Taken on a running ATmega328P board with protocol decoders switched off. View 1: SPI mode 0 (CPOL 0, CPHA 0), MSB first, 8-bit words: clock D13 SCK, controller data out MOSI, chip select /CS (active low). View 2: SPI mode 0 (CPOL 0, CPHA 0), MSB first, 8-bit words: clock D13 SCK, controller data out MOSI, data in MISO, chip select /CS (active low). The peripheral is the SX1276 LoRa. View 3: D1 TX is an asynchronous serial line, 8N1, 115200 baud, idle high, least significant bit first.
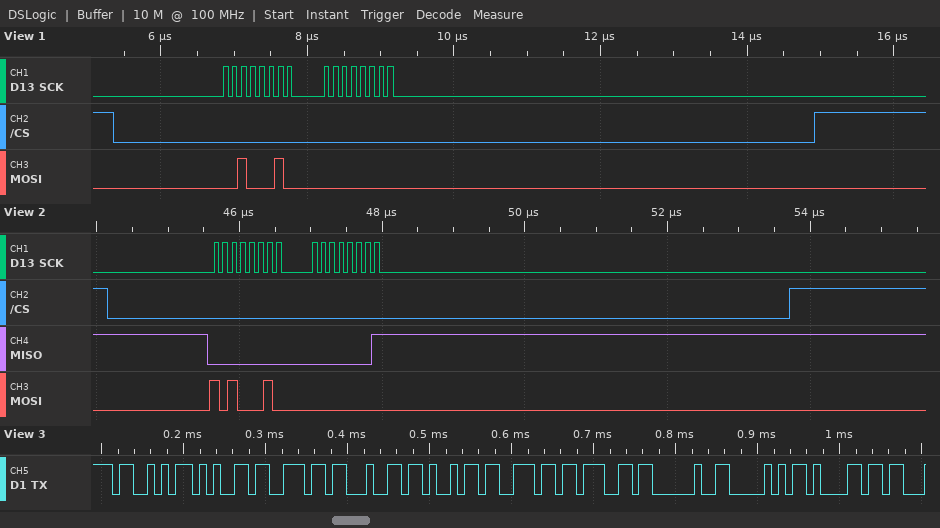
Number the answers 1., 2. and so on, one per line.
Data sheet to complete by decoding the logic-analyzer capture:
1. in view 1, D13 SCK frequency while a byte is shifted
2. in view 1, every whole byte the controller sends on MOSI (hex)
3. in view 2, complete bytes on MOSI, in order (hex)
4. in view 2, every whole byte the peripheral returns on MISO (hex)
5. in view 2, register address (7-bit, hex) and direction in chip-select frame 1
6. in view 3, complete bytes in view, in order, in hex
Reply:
1. 8 MHz
2. 0x22 0x00
3. A2 00
4. 00 01
5. 0x22 write
6. 53 65 6E 64 69 6E 67 20 50 61
